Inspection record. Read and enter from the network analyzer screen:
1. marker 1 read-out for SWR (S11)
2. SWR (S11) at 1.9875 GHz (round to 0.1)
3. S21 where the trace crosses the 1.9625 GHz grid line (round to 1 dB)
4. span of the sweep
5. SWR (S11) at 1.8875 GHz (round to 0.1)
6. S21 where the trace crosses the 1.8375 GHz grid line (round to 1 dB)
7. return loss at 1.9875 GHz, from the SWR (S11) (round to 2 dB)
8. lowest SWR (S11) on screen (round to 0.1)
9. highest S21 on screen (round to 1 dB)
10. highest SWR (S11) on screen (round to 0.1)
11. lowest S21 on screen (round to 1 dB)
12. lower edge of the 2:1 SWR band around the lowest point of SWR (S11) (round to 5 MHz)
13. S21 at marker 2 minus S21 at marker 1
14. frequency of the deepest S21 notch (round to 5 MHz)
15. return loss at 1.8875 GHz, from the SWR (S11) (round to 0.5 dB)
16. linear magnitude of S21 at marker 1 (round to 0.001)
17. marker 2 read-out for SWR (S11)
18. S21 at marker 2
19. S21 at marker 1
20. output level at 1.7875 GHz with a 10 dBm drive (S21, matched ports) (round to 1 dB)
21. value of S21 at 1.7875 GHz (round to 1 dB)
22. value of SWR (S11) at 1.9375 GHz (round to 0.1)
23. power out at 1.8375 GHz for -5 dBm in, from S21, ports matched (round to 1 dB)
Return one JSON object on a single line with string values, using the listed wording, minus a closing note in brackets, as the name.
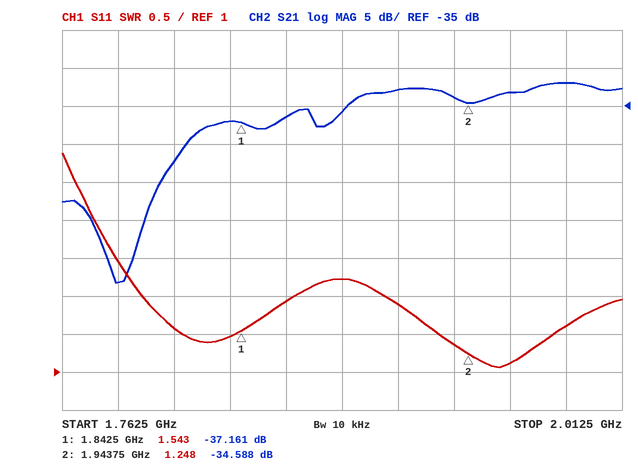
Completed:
{"marker 1 read-out for SWR": "1.543", "SWR (S11) at 1.9875 GHz": "1.6", "S21 where the trace crosses the 1.9625 GHz grid line": "-33 dB", "span of the sweep": "250 MHz", "SWR (S11) at 1.8875 GHz": "2.2", "S21 where the trace crosses the 1.8375 GHz grid line": "-37 dB", "return loss at 1.9875 GHz, from the SWR (S11)": "12 dB", "lowest SWR (S11) on screen": "1.1", "highest S21 on screen": "-32 dB", "highest SWR (S11) on screen": "3.9", "lowest S21 on screen": "-58 dB", "lower edge of the 2:1 SWR band around the lowest point of SWR (S11)": "1.905 GHz", "S21 at marker 2 minus S21 at marker 1": "2.573 dB", "frequency of the deepest S21 notch": "1.785 GHz", "return loss at 1.8875 GHz, from the SWR (S11)": "8.5 dB", "linear magnitude of S21 at marker 1": "0.014", "marker 2 read-out for SWR": "1.248", "S21 at marker 2": "-34.588 dB", "S21 at marker 1": "-37.161 dB", "output level at 1.7875 GHz with a 10 dBm drive (S21, matched ports)": "-48 dBm", "value of S21 at 1.7875 GHz": "-58 dB", "value of SWR (S11) at 1.9375 GHz": "1.4", "power out at 1.8375 GHz for -5 dBm in, from S21, ports matched": "-42 dBm"}
